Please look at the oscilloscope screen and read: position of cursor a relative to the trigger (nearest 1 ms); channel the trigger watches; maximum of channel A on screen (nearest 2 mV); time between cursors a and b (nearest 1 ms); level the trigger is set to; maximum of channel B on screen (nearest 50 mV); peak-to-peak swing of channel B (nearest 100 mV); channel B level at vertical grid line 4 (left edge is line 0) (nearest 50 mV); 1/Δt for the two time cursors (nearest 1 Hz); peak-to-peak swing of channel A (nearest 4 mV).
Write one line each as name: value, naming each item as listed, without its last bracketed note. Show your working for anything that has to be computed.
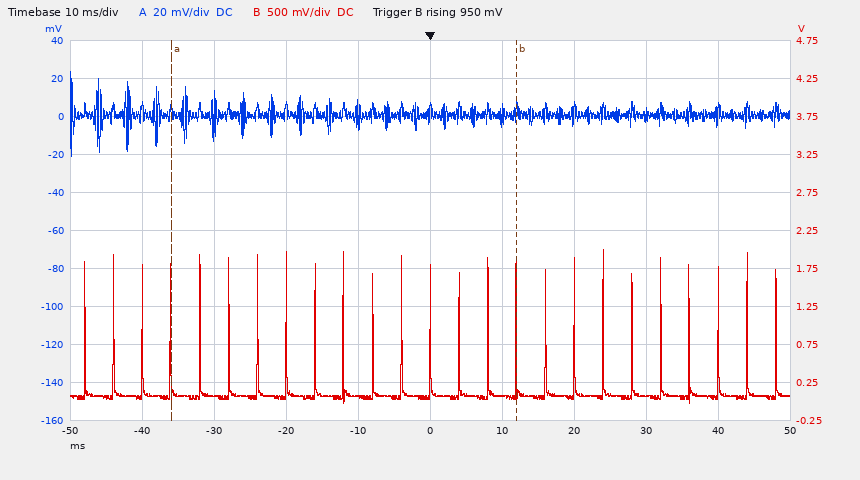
position of cursor a relative to the trigger: -36 ms
channel the trigger watches: channel B
maximum of channel A on screen: 24 mV
time between cursors a and b: 48 ms
level the trigger is set to: 950 mV
maximum of channel B on screen: 2.00 V
peak-to-peak swing of channel B: 2.00 V
channel B level at vertical grid line 4 (left edge is line 0): 50 mV
1/Δt for the two time cursors: 1 / 48 ms ≈ 21 Hz
peak-to-peak swing of channel A: 44 mV
